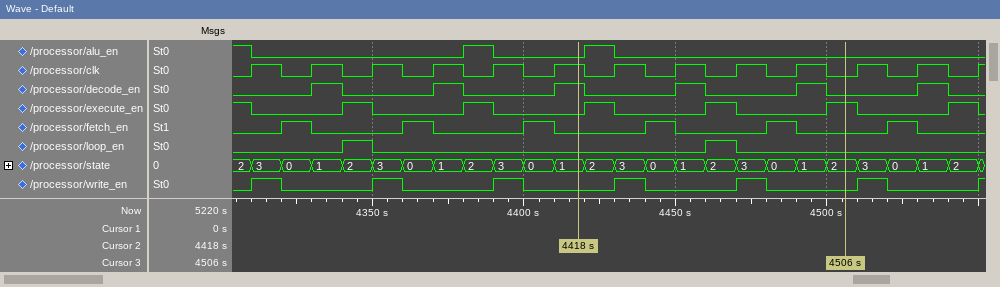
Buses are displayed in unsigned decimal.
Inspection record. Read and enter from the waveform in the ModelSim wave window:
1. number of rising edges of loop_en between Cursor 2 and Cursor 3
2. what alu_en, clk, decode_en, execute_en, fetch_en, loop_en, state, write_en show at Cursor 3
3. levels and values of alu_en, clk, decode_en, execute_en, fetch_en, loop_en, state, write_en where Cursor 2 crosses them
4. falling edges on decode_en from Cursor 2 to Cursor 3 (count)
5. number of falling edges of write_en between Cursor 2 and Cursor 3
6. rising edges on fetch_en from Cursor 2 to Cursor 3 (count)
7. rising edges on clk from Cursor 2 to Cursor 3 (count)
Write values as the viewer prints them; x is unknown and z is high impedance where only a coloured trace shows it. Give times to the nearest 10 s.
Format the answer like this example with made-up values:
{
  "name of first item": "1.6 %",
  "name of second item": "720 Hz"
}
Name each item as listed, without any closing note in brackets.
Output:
{
  "number of rising edges of loop_en between Cursor 2 and Cursor 3": "1",
  "what alu_en, clk, decode_en, execute_en, fetch_en, loop_en, state, write_en show at Cursor 3": "alu_en=0, clk=0, decode_en=0, execute_en=1, fetch_en=0, loop_en=0, state=2, write_en=0",
  "levels and values of alu_en, clk, decode_en, execute_en, fetch_en, loop_en, state, write_en where Cursor 2 crosses them": "alu_en=0, clk=1, decode_en=1, execute_en=0, fetch_en=0, loop_en=0, state=1, write_en=0",
  "falling edges on decode_en from Cursor 2 to Cursor 3": "3",
  "number of falling edges of write_en between Cursor 2 and Cursor 3": "2",
  "rising edges on fetch_en from Cursor 2 to Cursor 3": "2",
  "rising edges on clk from Cursor 2 to Cursor 3": "4"
}
